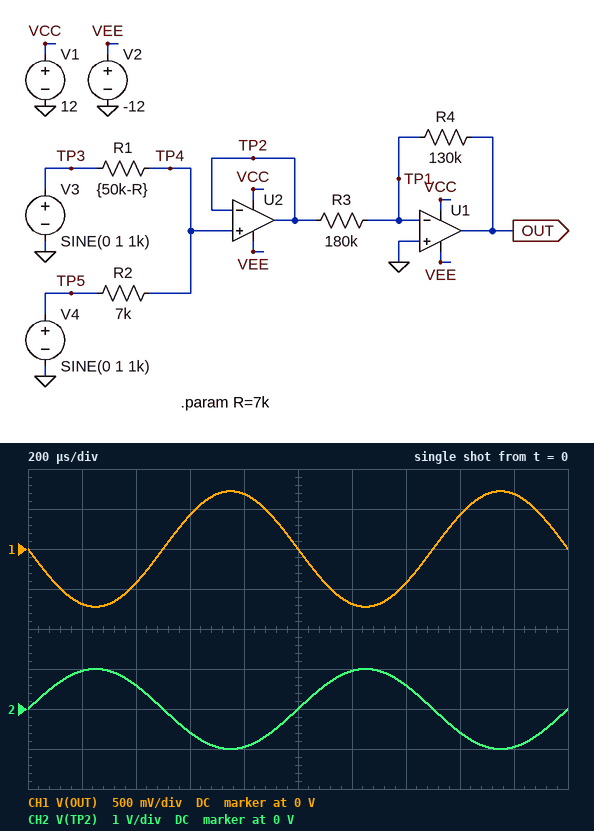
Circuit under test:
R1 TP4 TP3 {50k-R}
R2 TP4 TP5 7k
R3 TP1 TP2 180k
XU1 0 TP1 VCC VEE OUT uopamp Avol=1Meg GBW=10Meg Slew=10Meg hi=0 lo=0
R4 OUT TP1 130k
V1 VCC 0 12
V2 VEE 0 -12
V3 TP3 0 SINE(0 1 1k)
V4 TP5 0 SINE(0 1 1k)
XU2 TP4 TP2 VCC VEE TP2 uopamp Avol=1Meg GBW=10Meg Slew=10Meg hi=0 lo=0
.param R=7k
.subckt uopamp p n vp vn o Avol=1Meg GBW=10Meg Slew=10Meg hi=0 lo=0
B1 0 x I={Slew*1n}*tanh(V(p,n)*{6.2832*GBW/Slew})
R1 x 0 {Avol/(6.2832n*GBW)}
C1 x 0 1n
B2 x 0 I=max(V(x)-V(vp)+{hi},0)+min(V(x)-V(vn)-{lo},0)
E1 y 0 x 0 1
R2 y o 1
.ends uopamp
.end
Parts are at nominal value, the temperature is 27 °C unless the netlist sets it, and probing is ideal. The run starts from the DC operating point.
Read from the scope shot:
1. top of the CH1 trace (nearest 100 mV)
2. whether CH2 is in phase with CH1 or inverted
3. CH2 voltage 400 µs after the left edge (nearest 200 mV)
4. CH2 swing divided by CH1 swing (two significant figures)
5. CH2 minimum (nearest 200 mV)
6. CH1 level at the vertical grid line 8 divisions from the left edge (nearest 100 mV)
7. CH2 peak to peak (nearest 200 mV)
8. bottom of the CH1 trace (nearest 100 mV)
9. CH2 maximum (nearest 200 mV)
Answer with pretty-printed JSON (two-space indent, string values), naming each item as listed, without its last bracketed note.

{
  "top of the CH1 trace": "700 mV",
  "whether CH2 is in phase with CH1 or inverted": "inverted",
  "CH2 voltage 400 µs after the left edge": "600 mV",
  "CH2 swing divided by CH1 swing": "1.4",
  "CH2 minimum": "-1.0 V",
  "CH1 level at the vertical grid line 8 divisions from the left edge": "400 mV",
  "CH2 peak to peak": "2.0 V",
  "bottom of the CH1 trace": "-700 mV",
  "CH2 maximum": "1.0 V"
}
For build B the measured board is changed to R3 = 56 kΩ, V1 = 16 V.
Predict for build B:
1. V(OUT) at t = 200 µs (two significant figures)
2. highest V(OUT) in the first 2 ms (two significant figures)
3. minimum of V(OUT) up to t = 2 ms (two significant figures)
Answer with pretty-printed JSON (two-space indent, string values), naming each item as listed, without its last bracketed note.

{
  "V(OUT) at t = 200 µs": "-2.2 V",
  "highest V(OUT) in the first 2 ms": "2.3 V",
  "minimum of V(OUT) up to t = 2 ms": "-2.3 V"
}
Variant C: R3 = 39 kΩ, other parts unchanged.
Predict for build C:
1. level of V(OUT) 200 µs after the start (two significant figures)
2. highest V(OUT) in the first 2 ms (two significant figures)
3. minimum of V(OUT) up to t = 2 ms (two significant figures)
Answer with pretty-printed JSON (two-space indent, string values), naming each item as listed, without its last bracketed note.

{
  "level of V(OUT) 200 µs after the start": "-3.2 V",
  "highest V(OUT) in the first 2 ms": "3.3 V",
  "minimum of V(OUT) up to t = 2 ms": "-3.3 V"
}
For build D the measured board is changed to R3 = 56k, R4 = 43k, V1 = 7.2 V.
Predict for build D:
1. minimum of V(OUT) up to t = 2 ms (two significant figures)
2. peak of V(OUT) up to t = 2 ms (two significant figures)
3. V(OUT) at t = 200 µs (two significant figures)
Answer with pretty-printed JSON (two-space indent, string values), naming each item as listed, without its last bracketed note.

{
  "minimum of V(OUT) up to t = 2 ms": "-770 mV",
  "peak of V(OUT) up to t = 2 ms": "770 mV",
  "V(OUT) at t = 200 µs": "-730 mV"
}
